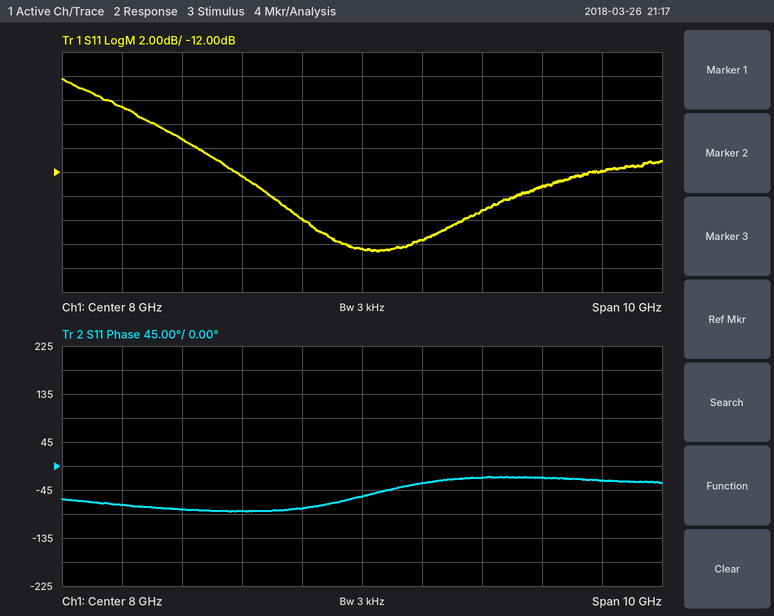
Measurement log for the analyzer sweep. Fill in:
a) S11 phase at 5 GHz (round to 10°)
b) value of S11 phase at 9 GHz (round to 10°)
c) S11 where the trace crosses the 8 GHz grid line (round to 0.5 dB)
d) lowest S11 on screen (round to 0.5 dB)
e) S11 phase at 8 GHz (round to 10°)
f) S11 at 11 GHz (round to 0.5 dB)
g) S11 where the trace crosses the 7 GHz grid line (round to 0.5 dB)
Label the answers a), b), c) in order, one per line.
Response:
a) -80°
b) -30°
c) -18.5 dB
d) -18.5 dB
e) -60°
f) -13.0 dB
g) -16.0 dB
